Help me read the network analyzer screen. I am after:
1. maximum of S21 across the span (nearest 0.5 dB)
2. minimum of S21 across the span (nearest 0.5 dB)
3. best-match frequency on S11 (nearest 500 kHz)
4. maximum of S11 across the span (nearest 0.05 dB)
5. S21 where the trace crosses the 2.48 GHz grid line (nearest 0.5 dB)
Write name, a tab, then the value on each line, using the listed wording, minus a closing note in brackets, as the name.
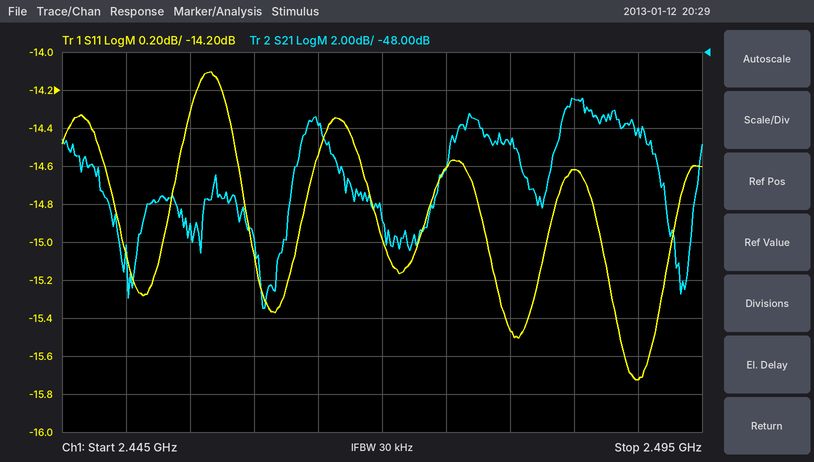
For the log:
maximum of S21 across the span	-50.5 dB
minimum of S21 across the span	-61.5 dB
best-match frequency on S11	2.4900 GHz
maximum of S11 across the span	-14.10 dB
S21 where the trace crosses the 2.48 GHz grid line	-53.0 dB
